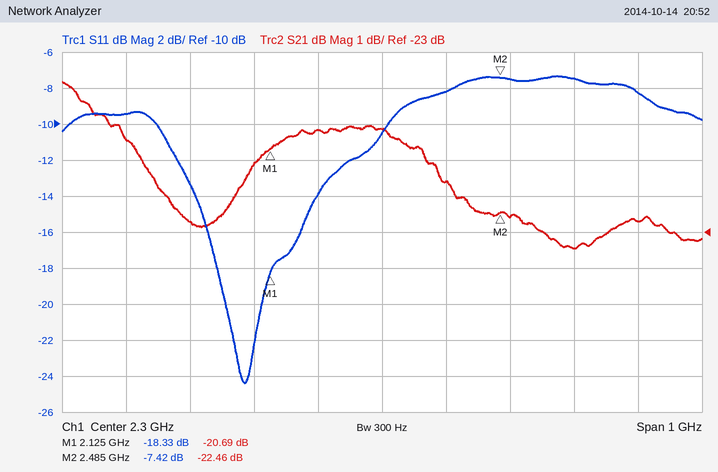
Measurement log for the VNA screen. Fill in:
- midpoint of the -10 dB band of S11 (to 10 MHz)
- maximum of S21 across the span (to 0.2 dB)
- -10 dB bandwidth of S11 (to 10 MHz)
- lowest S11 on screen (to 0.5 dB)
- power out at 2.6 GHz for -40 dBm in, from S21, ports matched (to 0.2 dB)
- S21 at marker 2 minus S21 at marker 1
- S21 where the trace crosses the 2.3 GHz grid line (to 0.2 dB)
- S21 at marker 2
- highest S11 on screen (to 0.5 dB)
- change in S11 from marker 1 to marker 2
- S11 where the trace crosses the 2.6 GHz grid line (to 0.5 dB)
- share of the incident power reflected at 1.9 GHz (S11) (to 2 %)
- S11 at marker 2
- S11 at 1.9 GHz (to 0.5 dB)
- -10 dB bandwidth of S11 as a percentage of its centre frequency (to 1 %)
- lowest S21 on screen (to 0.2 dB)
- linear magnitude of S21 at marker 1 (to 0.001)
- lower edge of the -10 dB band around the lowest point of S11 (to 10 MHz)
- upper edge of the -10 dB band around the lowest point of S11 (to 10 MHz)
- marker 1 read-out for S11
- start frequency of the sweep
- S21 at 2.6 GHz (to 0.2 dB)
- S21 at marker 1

2.13 GHz
-18.8 dB
360 MHz
-24.5 dB
-63.4 dBm
-1.77 dB
-20.2 dB
-22.46 dB
-7.5 dB
10.91 dB
-7.5 dB
12 %
-7.42 dB
-9.5 dB
17 %
-23.4 dB
0.092
1.95 GHz
2.31 GHz
-18.33 dB
1.8 GHz
-23.4 dB
-20.69 dB
